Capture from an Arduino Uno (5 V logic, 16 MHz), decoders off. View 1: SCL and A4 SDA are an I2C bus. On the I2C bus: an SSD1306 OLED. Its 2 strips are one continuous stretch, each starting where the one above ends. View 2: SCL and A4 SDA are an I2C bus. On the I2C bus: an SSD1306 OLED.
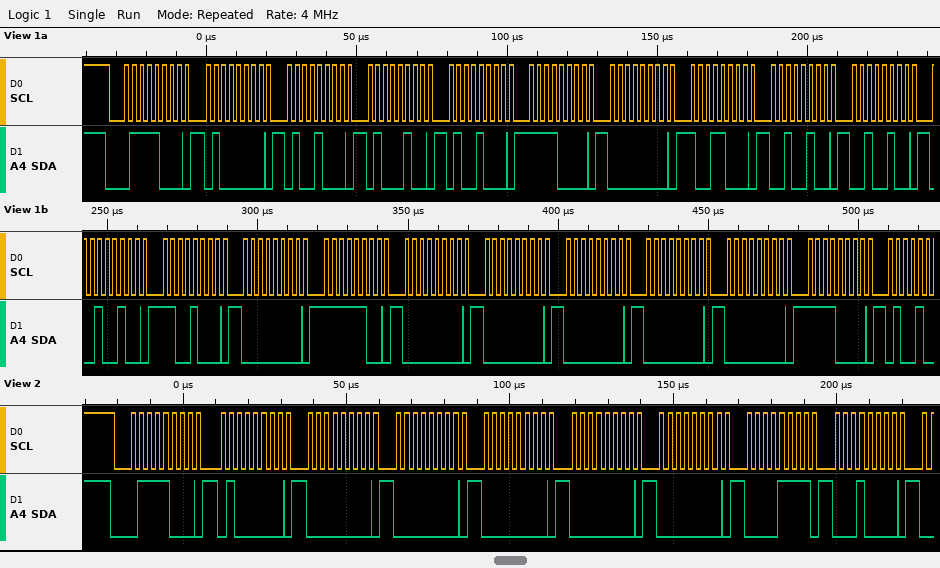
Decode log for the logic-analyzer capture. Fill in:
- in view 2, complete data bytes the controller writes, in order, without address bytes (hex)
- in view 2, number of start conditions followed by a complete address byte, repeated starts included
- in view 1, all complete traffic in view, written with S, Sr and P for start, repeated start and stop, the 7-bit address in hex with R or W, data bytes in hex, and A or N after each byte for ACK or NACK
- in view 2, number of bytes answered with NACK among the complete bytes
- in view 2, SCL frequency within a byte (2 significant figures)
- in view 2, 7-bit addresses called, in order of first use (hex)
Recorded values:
40 00 00 00 00 00 0F 10
1
S 3CW A 40 A 48 A 44 A 48 A F0 A 00 A 98 A 24 A 24 A 24 A C8 A 00 A FC A 00 A 00 A 00 A 00 A 00 A F0 A
0
400 kHz
0x3C
